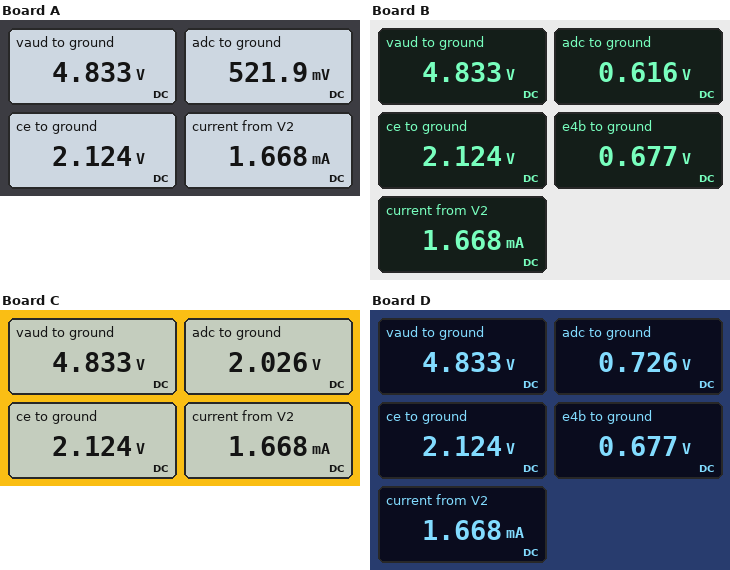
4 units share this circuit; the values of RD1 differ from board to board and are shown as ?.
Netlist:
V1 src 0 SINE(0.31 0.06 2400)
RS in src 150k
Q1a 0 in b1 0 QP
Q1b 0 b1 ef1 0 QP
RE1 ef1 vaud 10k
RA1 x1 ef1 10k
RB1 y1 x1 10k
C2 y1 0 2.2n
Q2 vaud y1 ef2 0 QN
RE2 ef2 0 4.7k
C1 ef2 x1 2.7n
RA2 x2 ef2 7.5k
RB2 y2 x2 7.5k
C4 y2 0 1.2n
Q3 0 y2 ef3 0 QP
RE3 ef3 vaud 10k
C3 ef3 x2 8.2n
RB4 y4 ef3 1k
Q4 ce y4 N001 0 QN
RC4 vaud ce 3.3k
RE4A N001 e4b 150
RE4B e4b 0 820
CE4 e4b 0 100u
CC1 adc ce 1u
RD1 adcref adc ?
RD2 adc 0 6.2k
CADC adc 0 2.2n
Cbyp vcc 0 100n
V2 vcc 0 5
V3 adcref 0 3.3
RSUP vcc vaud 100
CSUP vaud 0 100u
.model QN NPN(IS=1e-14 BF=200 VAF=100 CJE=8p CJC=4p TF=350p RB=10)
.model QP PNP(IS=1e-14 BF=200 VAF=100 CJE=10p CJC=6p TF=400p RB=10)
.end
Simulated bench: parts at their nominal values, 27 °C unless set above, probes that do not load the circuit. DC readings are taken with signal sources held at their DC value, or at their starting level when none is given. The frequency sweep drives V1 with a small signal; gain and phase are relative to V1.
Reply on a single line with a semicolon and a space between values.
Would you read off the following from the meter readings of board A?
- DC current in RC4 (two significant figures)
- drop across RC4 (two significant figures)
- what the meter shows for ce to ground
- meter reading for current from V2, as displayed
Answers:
820 µA; 2.7 V; 2.124 V; 1.668 mA
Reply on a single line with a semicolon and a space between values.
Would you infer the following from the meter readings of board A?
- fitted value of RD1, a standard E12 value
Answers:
33 kΩ
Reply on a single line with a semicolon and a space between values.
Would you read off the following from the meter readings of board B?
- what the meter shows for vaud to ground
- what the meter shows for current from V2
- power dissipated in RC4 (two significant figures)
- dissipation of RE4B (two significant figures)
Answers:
4.833 V; 1.668 mA; 2.2 mW; 560 µW
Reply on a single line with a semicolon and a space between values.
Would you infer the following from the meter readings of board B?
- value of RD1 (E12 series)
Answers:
27 kΩ
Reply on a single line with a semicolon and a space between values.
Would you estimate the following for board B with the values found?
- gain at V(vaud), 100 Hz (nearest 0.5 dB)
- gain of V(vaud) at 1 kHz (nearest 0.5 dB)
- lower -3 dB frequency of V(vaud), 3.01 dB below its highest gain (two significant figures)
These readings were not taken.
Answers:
-26.5 dB; -46.5 dB; 4.2 Hz
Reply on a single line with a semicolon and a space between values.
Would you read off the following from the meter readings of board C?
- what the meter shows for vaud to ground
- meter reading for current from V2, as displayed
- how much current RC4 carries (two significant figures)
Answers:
4.833 V; 1.668 mA; 820 µA
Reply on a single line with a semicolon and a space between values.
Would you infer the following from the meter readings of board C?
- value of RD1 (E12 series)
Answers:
3.9 kΩ
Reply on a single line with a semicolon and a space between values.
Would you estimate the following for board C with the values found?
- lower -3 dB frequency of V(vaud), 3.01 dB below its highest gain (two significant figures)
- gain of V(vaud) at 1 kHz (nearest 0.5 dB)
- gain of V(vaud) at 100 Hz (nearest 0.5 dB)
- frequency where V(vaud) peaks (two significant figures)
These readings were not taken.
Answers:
4.4 Hz; -49.5 dB; -28.5 dB; 11 Hz
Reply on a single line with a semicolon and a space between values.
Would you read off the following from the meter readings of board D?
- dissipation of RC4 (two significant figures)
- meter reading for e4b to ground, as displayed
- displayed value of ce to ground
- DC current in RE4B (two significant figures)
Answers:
2.2 mW; 0.677 V; 2.124 V; 830 µA
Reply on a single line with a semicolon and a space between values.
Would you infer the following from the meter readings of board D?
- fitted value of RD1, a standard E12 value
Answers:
22 kΩ
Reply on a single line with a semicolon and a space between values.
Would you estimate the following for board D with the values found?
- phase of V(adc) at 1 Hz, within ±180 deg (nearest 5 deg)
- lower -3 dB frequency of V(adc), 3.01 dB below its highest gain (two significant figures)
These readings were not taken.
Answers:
-70 deg; 24 Hz
